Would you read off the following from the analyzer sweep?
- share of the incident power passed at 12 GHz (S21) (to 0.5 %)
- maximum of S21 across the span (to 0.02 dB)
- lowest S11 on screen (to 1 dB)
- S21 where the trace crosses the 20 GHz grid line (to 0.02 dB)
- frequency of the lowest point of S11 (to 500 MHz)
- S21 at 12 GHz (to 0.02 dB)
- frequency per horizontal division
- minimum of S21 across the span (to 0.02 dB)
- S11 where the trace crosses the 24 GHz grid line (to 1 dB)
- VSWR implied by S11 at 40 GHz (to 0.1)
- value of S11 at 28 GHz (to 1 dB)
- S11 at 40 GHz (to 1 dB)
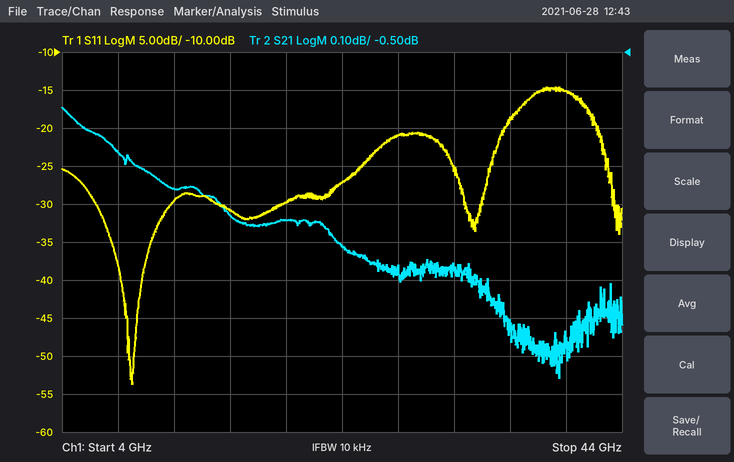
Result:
82.0 %
-0.64 dB
-54 dB
-0.94 dB
9.0 GHz
-0.86 dB
4 GHz
-1.36 dB
-27 dB
1.4
-21 dB
-15 dB
